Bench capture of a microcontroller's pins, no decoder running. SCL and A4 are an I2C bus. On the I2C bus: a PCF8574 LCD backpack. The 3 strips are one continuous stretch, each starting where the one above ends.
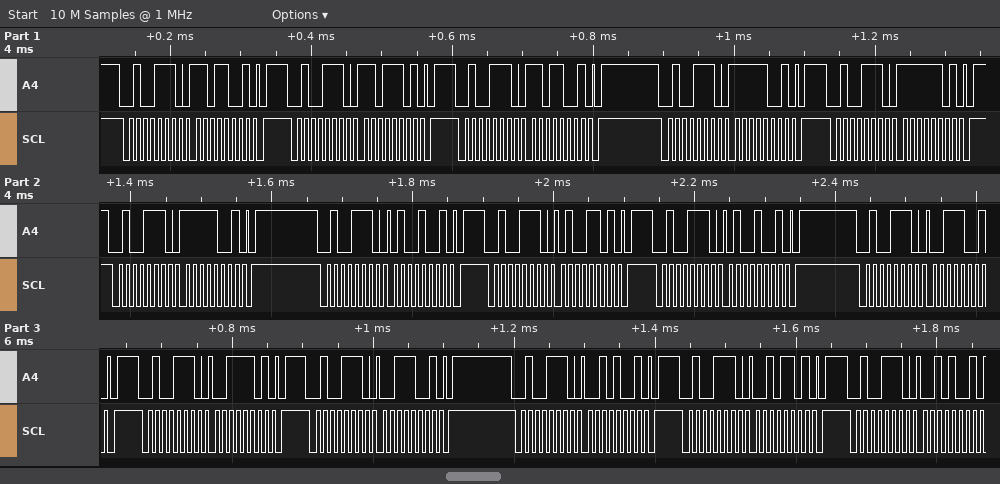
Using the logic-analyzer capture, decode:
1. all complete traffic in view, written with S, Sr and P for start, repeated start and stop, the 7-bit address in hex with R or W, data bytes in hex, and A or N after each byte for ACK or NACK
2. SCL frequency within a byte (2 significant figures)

S 27W A D9 A P S 27W A DD A P S 27W A D9 A P S 27W A F9 A P S 27W A FD A P S 27W A F9 A P S 27W A 49 A P S 27W A 4D A P S 27W A 49 A P S 27W A 39 A P S 27W A 3D A P S 27W A 39 A P S 27W A 29 A P S 27W A 2D A P S 27W A 29 A
100 kHz
